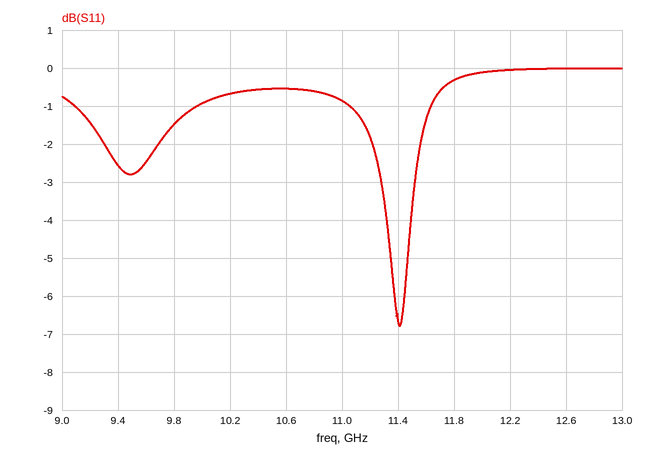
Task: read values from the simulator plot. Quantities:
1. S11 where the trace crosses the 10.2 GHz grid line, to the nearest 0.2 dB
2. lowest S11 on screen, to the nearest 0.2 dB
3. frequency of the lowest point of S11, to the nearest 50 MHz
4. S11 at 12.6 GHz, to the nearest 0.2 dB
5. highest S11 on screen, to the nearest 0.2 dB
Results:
-0.6 dB
-6.8 dB
11.40 GHz
0.0 dB
0.0 dB
